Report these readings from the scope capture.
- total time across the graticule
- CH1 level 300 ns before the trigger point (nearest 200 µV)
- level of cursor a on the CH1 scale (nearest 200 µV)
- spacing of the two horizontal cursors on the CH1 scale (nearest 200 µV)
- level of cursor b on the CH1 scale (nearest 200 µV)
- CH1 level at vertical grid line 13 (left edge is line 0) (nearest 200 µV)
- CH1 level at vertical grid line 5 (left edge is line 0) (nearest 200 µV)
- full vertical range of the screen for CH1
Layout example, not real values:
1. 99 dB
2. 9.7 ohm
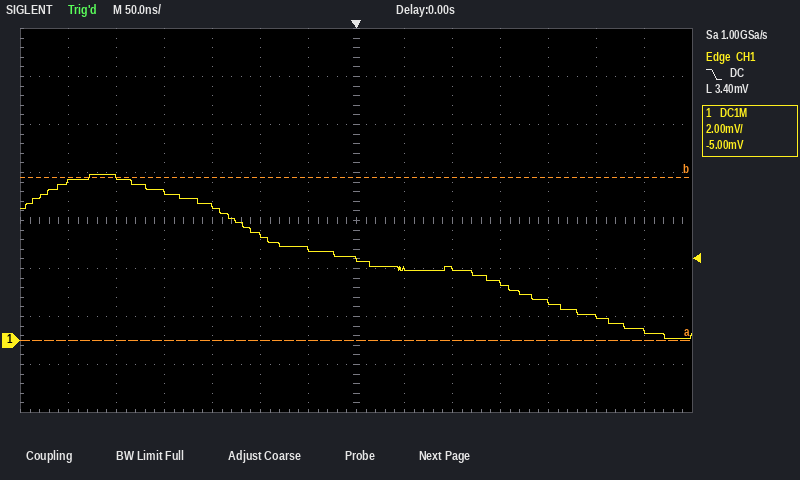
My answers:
1. 700 ns
2. 6.6 mV
3. 0.0 mV
4. 6.8 mV
5. 6.8 mV
6. 400 µV
7. 4.4 mV
8. 16 mV
